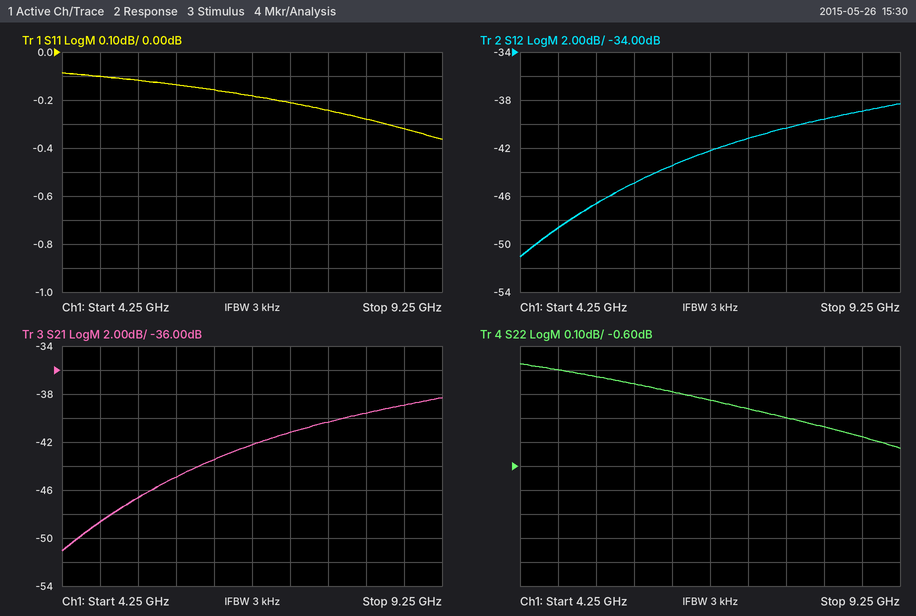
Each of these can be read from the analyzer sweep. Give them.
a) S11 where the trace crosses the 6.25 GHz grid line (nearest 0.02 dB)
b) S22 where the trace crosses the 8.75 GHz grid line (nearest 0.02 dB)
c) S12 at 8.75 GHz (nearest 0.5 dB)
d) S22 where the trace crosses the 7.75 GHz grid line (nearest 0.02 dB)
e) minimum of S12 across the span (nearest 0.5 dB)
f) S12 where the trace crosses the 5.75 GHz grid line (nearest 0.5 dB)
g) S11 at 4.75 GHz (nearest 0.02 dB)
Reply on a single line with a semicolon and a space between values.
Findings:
-0.16 dB; -0.48 dB; -39.0 dB; -0.40 dB; -51.0 dB; -45.0 dB; -0.10 dB
